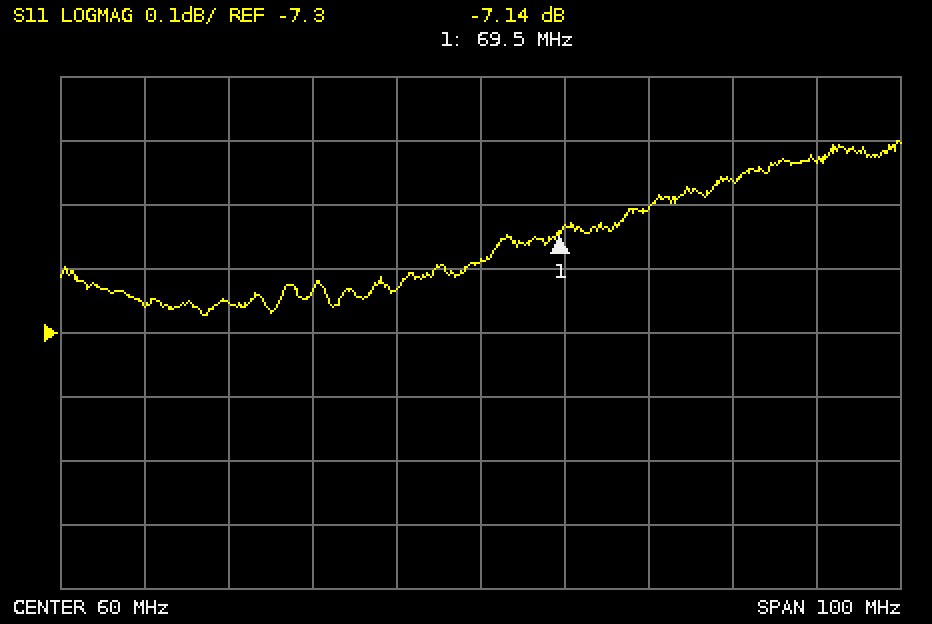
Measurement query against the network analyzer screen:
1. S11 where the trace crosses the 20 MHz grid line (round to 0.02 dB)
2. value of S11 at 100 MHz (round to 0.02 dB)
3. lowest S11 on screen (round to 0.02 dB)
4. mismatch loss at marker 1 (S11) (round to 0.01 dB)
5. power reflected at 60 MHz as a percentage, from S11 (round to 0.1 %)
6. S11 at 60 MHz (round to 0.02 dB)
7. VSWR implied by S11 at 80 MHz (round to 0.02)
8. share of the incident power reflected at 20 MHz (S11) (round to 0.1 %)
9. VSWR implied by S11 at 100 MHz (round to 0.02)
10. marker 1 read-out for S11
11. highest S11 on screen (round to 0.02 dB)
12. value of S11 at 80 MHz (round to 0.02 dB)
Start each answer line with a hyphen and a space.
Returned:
- -7.26 dB
- -7.04 dB
- -7.28 dB
- 0.93 dB
- 19.1 %
- -7.18 dB
- 2.58
- 18.8 %
- 2.60
- -7.14 dB
- -7.00 dB
- -7.10 dB
